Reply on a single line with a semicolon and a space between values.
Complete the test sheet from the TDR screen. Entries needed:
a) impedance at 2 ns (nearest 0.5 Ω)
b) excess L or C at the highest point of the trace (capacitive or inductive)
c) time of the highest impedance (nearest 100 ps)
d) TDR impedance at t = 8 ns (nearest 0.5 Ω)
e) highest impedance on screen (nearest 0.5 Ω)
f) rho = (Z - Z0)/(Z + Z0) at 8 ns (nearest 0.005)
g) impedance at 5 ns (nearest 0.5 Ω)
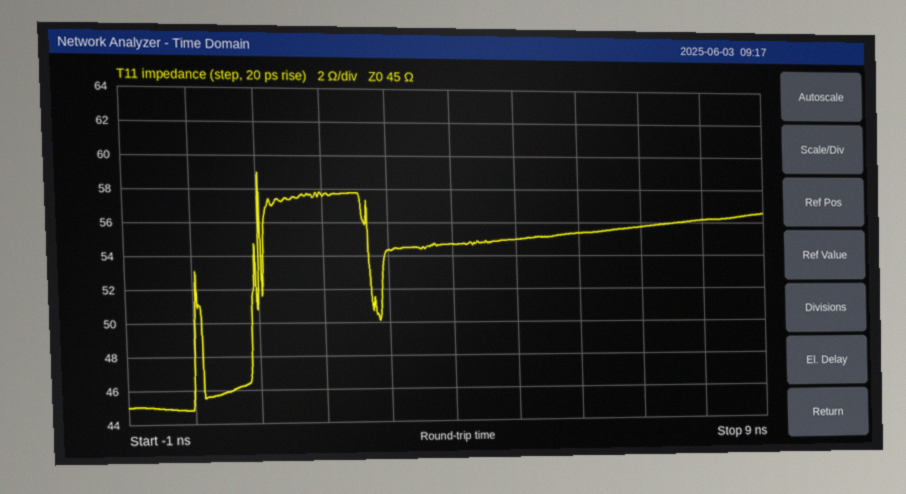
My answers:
57.5 Ω; inductive; 1.0 ns; 56.0 Ω; 59.0 Ω; +0.110; 55.0 Ω
